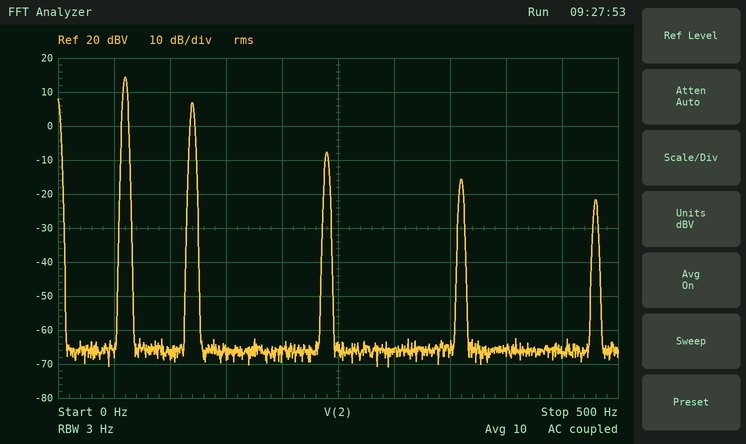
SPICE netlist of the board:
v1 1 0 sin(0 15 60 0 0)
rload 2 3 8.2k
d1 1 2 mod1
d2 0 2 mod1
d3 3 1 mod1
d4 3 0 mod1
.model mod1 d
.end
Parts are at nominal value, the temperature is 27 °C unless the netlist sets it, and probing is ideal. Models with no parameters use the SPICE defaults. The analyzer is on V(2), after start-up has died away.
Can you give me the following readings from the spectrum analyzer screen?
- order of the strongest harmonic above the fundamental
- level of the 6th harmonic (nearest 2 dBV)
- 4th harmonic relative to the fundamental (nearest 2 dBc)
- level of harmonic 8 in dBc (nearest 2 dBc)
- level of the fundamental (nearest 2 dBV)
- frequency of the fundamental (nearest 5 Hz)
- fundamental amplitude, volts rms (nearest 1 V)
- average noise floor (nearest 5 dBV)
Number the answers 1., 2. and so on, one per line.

1. 2
2. -16 dBV
3. -22 dBc
4. -36 dBc
5. 14 dBV
6. 60 Hz
7. 5 V
8. -65 dBV
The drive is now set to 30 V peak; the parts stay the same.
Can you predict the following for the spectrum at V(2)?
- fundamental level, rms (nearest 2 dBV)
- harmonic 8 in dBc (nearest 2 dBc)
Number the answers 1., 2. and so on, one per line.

1. 20 dBV
2. -34 dBc
